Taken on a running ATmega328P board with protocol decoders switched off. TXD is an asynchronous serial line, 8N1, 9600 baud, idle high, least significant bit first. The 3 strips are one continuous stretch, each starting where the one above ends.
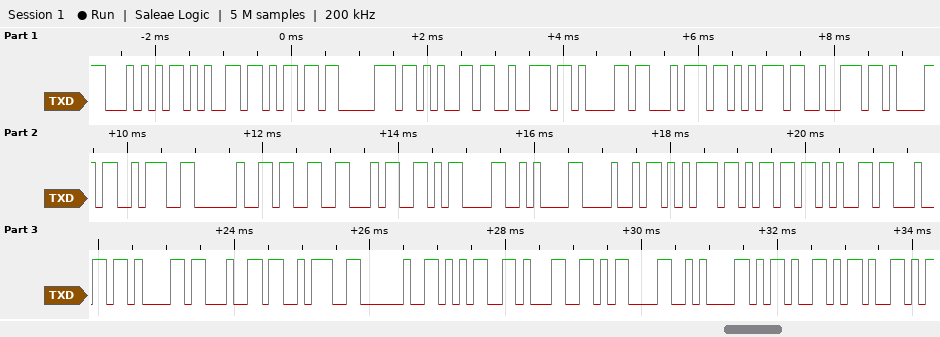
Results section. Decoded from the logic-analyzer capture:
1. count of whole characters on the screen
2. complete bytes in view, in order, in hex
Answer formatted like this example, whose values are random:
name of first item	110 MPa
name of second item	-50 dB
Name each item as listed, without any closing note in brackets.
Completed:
count of whole characters on the screen	32
complete bytes in view, in order, in hex	54 65 6D 70 65 72 61 74 75 72 61 3A 20 33 34 0D 0A 48 75 6D 65 64 61 64 3A 20 35 31 0D 0A 2D 2D
